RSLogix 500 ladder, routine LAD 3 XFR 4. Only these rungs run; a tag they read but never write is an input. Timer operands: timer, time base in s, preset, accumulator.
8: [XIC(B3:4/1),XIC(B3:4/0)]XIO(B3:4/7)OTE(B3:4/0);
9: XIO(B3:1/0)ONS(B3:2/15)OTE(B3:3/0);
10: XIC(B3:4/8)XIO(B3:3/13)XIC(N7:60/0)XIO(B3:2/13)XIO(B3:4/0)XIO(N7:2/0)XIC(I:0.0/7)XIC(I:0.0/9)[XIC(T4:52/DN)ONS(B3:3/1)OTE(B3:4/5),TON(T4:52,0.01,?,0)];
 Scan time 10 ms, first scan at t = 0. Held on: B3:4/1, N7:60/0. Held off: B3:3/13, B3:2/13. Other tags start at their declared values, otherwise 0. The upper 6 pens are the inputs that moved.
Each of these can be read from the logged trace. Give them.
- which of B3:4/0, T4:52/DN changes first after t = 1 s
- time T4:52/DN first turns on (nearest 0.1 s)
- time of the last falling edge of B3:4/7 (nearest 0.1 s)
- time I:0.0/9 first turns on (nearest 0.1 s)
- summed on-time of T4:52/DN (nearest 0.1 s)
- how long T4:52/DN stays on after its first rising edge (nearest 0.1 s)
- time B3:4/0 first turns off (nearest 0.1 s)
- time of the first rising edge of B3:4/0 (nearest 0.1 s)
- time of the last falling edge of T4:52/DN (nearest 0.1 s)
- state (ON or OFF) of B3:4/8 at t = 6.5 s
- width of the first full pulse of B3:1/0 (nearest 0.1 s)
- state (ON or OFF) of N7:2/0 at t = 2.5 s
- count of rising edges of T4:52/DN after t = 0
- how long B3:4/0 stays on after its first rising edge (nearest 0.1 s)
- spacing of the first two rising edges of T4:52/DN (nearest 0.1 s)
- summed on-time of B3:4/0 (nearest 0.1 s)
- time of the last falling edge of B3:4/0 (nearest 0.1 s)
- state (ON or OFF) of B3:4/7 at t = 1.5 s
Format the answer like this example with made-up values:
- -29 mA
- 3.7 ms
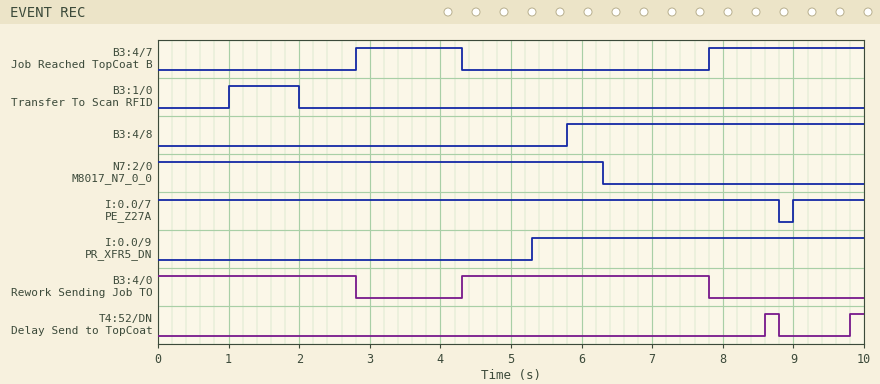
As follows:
- B3:4/0
- 8.6 s
- 4.3 s
- 5.3 s
- 0.4 s
- 0.2 s
- 2.8 s
- 4.3 s
- 8.8 s
- ON
- 1.0 s
- ON
- 2
- 3.5 s
- 1.2 s
- 6.3 s
- 7.8 s
- OFF
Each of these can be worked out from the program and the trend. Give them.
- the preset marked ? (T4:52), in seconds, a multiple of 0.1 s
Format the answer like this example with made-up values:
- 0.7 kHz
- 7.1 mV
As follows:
- 0.8 s
